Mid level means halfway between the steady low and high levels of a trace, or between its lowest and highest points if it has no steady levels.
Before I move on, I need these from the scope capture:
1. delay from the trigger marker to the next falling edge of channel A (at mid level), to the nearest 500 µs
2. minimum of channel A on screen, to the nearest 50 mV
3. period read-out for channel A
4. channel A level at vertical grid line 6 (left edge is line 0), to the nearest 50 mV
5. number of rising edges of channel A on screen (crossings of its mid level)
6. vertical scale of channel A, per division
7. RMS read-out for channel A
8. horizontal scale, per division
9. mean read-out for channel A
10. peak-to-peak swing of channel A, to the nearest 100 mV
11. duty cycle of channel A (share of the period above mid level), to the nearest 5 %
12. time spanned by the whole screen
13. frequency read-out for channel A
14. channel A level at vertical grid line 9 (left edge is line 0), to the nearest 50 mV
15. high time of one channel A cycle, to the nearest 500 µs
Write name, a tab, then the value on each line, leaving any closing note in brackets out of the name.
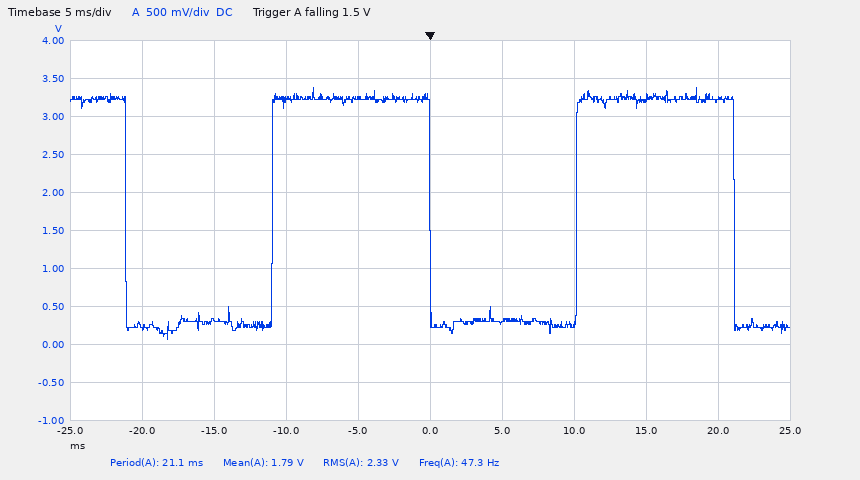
delay from the trigger marker to the next falling edge of channel A (at mid level), to the nearest 500 µs	21.0 ms
minimum of channel A on screen, to the nearest 50 mV	50 mV
period read-out for channel A	21.1 ms
channel A level at vertical grid line 6 (left edge is line 0), to the nearest 50 mV	300 mV
number of rising edges of channel A on screen	2
vertical scale of channel A, per division	500 mV
RMS read-out for channel A	2.33 V
horizontal scale, per division	5 ms
mean read-out for channel A	1.79 V
peak-to-peak swing of channel A, to the nearest 100 mV	3.30 V
duty cycle of channel A (share of the period above mid level), to the nearest 5 %	50 %
time spanned by the whole screen	50 ms
frequency read-out for channel A	47.3 Hz
channel A level at vertical grid line 9 (left edge is line 0), to the nearest 50 mV	3.20 V
high time of one channel A cycle, to the nearest 500 µs	11.0 ms
